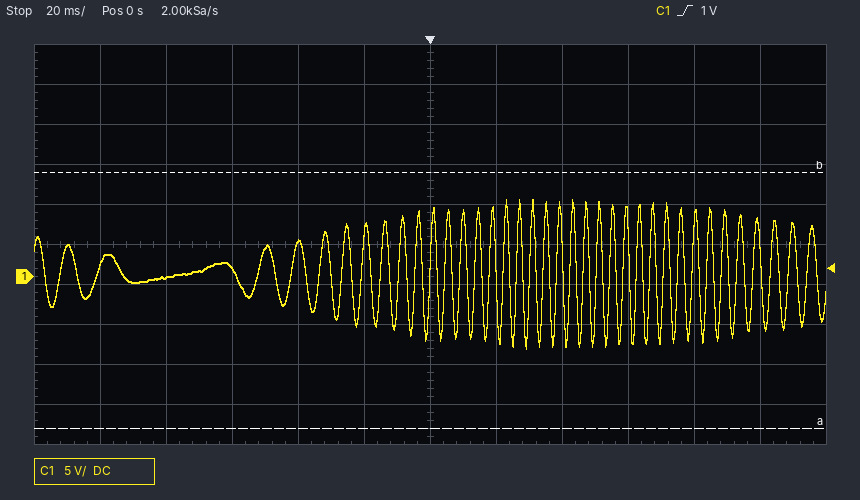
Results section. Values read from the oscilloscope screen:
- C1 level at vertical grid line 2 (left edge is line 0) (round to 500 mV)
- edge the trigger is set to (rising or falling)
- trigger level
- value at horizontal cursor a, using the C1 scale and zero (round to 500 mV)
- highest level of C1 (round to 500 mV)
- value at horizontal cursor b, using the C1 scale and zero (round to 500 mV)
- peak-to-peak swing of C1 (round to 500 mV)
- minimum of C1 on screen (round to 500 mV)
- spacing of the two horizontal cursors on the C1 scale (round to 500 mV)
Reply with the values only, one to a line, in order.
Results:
0.0 V
rising
1 V
-19.0 V
9.5 V
13.0 V
18.5 V
-9.0 V
32.0 V
